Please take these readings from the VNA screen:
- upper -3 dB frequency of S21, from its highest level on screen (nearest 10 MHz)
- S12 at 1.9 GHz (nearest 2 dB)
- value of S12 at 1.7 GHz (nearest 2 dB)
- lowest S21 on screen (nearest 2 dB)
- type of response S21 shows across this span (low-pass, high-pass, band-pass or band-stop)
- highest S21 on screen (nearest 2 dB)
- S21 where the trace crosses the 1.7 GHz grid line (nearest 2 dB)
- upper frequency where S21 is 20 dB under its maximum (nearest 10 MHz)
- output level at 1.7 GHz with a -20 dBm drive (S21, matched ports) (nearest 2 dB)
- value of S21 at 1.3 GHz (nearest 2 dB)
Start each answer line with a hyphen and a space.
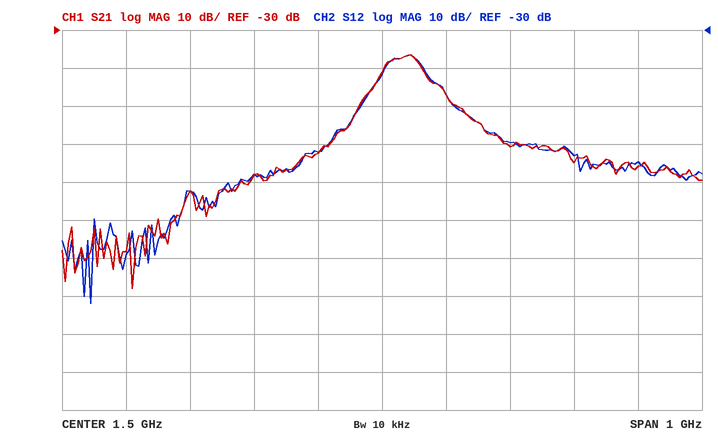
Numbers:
- 1.56 GHz
- -64 dB
- -60 dB
- -98 dB
- band-pass
- -36 dB
- -60 dB
- 1.66 GHz
- -80 dBm
- -68 dB
